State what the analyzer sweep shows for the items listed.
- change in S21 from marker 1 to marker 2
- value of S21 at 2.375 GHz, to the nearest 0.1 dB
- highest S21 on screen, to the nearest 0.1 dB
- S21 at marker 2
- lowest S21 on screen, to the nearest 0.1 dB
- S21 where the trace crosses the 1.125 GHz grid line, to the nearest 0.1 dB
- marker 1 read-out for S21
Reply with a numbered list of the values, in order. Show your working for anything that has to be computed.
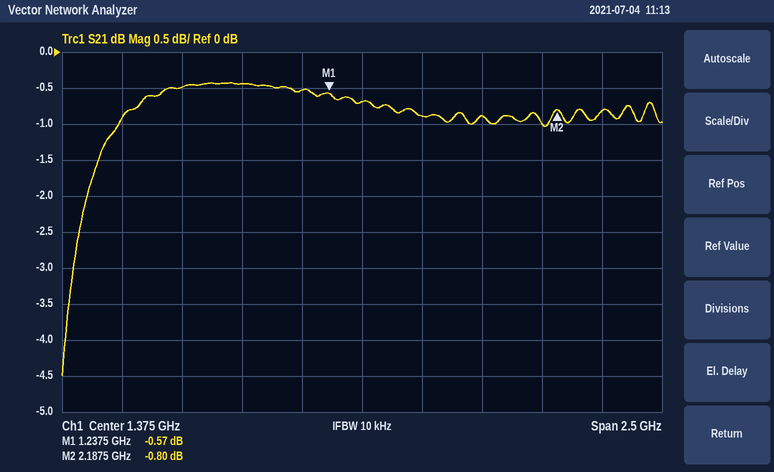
1. -0.8 − (-0.57) = -0.23 dB
2. -0.8 dB
3. -0.4 dB
4. -0.80 dB
5. -4.5 dB
6. -0.5 dB
7. -0.57 dB
